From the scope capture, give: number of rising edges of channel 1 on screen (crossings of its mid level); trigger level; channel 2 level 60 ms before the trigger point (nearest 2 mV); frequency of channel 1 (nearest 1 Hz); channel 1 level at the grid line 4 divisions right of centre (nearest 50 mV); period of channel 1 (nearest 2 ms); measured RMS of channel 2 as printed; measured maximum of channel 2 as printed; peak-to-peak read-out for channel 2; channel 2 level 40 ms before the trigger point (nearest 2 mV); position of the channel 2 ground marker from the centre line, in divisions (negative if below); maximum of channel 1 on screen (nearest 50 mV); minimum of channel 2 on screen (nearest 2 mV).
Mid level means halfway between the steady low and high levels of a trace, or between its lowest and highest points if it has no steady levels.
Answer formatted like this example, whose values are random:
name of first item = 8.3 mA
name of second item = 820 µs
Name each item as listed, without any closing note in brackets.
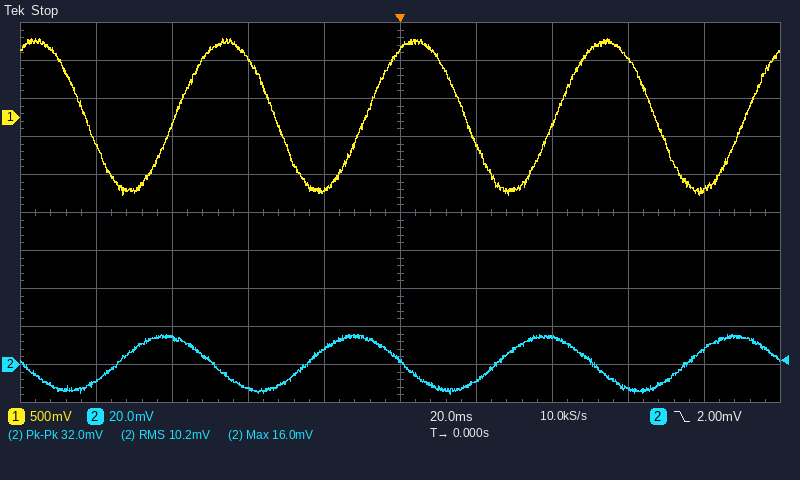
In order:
number of rising edges of channel 1 on screen = 4
trigger level = 2.00 mV
channel 2 level 60 ms before the trigger point = 14 mV
frequency of channel 1 = 20 Hz
channel 1 level at the grid line 4 divisions right of centre = -950 mV
period of channel 1 = 50 ms
measured RMS of channel 2 as printed = 10.2 mV
measured maximum of channel 2 as printed = 16.0 mV
peak-to-peak read-out for channel 2 = 32.0 mV
channel 2 level 40 ms before the trigger point = -14 mV
position of the channel 2 ground marker from the centre line, in divisions = -4.0 div
maximum of channel 1 on screen = 1.05 V
minimum of channel 2 on screen = -16 mV
